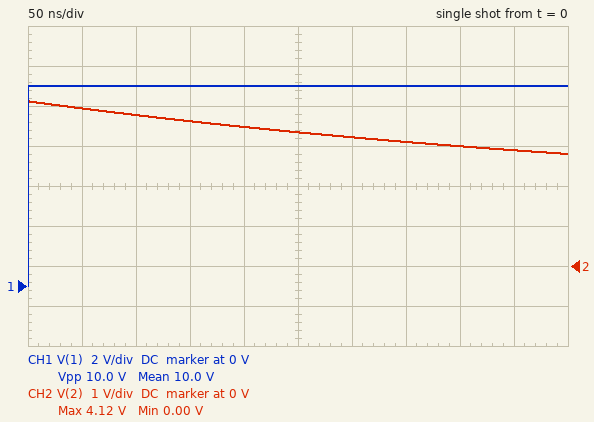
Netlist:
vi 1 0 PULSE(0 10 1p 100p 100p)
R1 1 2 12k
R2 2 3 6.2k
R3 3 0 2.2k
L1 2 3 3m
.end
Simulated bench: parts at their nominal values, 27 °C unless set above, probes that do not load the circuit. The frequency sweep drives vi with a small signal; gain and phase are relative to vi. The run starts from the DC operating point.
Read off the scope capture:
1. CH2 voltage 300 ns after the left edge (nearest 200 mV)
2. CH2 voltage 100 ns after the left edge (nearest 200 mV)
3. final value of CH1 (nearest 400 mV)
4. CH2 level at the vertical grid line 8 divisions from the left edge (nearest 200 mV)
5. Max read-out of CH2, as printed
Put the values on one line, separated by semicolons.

3.2 V; 3.8 V; 10.0 V; 3.0 V; 4.12 V
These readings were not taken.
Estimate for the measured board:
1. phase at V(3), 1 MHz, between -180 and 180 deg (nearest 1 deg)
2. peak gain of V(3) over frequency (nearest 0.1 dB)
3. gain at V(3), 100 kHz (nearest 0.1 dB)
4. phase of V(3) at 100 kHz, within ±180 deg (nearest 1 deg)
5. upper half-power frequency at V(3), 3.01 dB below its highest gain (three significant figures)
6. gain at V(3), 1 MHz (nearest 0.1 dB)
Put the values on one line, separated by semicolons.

-5 deg; -16.2 dB; -16.6 dB; -7 deg; 1.30 MHz; -19.1 dB
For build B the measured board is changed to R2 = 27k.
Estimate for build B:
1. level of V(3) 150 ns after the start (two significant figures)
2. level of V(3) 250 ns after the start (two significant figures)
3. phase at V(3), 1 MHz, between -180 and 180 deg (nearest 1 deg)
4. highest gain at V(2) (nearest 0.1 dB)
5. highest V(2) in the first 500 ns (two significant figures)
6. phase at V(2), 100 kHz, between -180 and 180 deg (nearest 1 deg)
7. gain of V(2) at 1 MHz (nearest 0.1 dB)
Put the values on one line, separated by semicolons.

910 mV; 1.1 V; -29 deg; -3.0 dB; 7.1 V; 31 deg; -3.9 dB
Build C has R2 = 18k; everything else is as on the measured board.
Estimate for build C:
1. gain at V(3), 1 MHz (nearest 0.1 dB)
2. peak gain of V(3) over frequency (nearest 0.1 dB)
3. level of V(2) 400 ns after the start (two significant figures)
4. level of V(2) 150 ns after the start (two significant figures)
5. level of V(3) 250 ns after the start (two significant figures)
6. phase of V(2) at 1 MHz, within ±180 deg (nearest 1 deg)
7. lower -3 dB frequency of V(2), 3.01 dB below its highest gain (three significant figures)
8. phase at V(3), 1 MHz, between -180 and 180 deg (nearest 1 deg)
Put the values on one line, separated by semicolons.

-21.2 dB; -16.2 dB; 3.2 V; 4.7 V; 1.1 V; 17 deg; 395 kHz; -21 deg
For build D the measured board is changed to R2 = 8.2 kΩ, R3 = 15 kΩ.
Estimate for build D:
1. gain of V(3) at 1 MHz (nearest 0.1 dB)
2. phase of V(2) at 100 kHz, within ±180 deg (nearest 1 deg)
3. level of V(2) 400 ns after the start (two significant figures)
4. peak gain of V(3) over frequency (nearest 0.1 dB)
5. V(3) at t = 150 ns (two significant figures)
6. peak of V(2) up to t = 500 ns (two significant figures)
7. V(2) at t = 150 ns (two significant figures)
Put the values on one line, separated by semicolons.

-7.1 dB; 3 deg; 6.0 V; -5.1 dB; 4.6 V; 6.6 V; 6.3 V
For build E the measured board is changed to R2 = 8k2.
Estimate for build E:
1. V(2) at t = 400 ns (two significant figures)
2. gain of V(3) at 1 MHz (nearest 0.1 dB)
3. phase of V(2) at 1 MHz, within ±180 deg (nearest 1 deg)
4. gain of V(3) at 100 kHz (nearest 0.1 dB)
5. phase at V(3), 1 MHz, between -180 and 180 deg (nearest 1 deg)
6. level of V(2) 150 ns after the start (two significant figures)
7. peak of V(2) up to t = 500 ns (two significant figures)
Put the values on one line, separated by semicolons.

3.1 V; -19.7 dB; 10 deg; -16.5 dB; -8 deg; 3.9 V; 4.6 V
